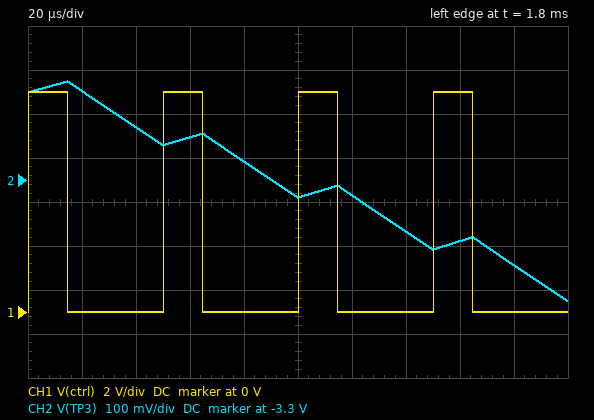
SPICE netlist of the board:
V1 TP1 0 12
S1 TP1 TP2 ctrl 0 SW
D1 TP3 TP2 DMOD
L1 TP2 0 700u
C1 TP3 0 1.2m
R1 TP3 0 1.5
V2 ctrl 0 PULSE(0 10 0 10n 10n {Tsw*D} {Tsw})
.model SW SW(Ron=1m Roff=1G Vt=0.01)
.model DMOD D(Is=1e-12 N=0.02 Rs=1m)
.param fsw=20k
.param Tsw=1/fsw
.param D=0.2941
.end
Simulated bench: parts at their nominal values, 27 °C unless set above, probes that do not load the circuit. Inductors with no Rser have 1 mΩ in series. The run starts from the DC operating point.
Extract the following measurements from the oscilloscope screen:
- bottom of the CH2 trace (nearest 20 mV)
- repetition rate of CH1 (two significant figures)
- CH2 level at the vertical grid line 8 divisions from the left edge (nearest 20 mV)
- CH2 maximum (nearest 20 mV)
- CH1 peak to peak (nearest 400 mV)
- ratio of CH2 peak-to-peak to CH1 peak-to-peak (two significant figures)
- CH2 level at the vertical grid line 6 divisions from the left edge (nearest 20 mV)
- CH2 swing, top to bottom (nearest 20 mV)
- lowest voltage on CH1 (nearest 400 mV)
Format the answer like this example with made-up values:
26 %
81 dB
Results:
-3.58 V
20 kHz
-3.44 V
-3.08 V
10.0 V
0.050
-3.34 V
500 mV
0 V
